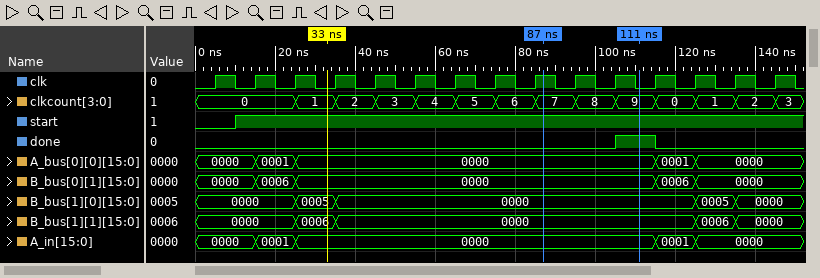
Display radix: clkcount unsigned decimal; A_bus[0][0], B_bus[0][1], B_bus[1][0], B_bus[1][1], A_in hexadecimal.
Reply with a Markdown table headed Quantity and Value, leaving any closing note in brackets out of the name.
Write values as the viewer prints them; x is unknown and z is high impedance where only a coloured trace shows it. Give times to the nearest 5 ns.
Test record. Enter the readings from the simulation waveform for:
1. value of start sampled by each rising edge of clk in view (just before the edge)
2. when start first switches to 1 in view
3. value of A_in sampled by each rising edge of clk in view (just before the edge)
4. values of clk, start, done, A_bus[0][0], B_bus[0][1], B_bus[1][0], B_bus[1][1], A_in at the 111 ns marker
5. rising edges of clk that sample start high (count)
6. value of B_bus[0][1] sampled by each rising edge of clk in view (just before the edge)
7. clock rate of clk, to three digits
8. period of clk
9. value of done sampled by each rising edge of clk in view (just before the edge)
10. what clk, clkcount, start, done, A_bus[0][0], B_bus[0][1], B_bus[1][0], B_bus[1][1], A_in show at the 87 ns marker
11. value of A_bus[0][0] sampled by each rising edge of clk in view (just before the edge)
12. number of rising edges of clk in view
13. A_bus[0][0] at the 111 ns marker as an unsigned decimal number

| Quantity | Value |
|---|---|
| value of start sampled by each rising edge of clk in view | 0 1 1 1 1 1 1 1 1 1 1 1 1 1 1 |
| when start first switches to 1 in view | 10 ns |
| value of A_in sampled by each rising edge of clk in view | 0000, 0000, 0001, 0000, 0000, 0000, 0000, 0000, 0000, 0000, 0000, 0000, 0001, 0000, 0000 |
| values of clk, start, done, A_bus[0][0], B_bus[0][1], B_bus[1][0], B_bus[1][1], A_in at the 111 ns marker | clk=0, start=1, done=1, A_bus[0][0]=0000, B_bus[0][1]=0000, B_bus[1][0]=0000, B_bus[1][1]=0000, A_in=0000 |
| rising edges of clk that sample start high | 14 |
| value of B_bus[0][1] sampled by each rising edge of clk in view | 0000, 0000, 0006, 0000, 0000, 0000, 0000, 0000, 0000, 0000, 0000, 0000, 0006, 0000, 0000 |
| clock rate of clk, to three digits | 100 MHz |
| period of clk | 10 ns |
| value of done sampled by each rising edge of clk in view | 0 0 0 0 0 0 0 0 0 0 0 1 0 0 0 |
| what clk, clkcount, start, done, A_bus[0][0], B_bus[0][1], B_bus[1][0], B_bus[1][1], A_in show at the 87 ns marker | clk=1, clkcount=7, start=1, done=0, A_bus[0][0]=0000, B_bus[0][1]=0000, B_bus[1][0]=0000, B_bus[1][1]=0000, A_in=0000 |
| value of A_bus[0][0] sampled by each rising edge of clk in view | 0000, 0000, 0001, 0000, 0000, 0000, 0000, 0000, 0000, 0000, 0000, 0000, 0001, 0000, 0000 |
| number of rising edges of clk in view | 15 |
| A_bus[0][0] at the 111 ns marker as an unsigned decimal number | 0 |
